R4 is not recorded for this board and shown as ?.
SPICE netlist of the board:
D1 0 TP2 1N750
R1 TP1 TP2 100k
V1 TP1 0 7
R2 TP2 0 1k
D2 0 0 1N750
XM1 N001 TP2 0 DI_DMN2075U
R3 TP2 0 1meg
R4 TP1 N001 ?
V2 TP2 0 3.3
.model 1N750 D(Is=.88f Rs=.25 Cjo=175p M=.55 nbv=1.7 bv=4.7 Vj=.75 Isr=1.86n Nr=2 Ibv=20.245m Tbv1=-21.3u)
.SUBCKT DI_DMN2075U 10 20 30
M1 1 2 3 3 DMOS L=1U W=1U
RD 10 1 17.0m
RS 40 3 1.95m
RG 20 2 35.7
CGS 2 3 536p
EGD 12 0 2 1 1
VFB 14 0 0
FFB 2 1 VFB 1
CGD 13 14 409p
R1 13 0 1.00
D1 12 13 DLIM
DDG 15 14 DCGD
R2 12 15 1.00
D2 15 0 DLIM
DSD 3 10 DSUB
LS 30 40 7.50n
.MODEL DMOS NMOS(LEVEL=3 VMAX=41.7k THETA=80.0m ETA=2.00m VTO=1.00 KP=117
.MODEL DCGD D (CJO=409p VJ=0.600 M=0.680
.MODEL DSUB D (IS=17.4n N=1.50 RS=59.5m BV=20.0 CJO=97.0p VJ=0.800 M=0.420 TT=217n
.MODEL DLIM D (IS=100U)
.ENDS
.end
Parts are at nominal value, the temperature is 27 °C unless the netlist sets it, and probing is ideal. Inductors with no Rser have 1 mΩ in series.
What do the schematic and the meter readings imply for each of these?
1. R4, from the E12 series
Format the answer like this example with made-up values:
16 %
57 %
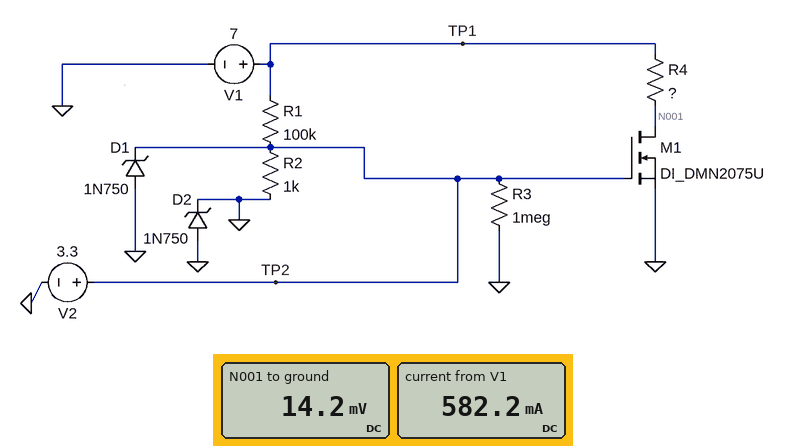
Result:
12 Ω
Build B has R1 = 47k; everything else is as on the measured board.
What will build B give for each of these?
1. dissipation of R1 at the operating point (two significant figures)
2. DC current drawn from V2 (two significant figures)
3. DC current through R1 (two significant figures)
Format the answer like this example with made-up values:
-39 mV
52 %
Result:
290 µW
3.2 mA
79 µA
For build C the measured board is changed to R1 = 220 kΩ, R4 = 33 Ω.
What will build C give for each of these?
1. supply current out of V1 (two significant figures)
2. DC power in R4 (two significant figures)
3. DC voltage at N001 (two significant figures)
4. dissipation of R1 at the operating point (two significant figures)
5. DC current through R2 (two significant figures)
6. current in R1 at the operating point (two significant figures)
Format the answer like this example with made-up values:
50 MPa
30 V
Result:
210 mA
1.5 W
5.2 mV
62 µW
3.3 mA
17 µA
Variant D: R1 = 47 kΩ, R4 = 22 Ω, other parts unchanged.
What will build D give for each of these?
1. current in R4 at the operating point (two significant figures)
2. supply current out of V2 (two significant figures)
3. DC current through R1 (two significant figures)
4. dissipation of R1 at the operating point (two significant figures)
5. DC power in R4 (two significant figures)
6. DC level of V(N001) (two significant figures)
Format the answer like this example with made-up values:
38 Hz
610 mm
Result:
320 mA
3.2 mA
79 µA
290 µW
2.2 W
7.7 mV
